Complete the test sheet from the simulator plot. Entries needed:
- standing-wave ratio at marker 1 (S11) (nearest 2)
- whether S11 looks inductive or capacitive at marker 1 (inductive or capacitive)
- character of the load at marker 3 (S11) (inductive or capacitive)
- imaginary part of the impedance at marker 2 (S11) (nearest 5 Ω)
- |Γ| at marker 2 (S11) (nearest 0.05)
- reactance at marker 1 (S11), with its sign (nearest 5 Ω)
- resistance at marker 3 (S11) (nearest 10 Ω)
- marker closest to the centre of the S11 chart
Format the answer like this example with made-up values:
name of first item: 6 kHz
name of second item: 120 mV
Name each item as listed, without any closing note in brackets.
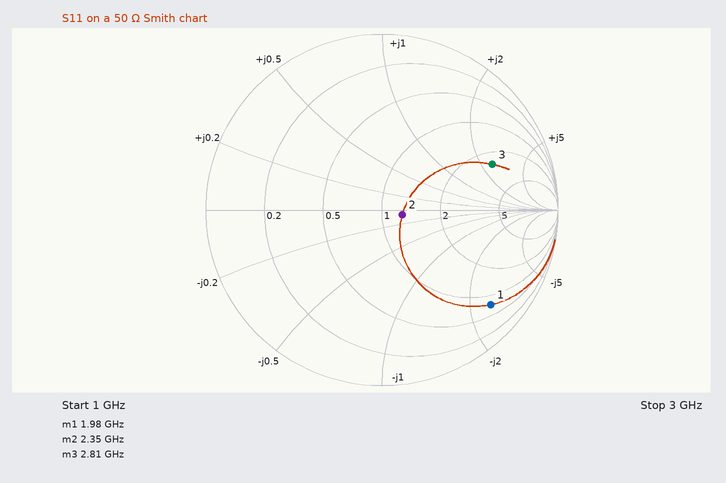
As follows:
standing-wave ratio at marker 1 (S11): 10
whether S11 looks inductive or capacitive at marker 1: capacitive
character of the load at marker 3 (S11): inductive
imaginary part of the impedance at marker 2 (S11): -5 Ω
|Γ| at marker 2 (S11): 0.10
reactance at marker 1 (S11), with its sign: -125 Ω
resistance at marker 3 (S11): 130 Ω
marker closest to the centre of the S11 chart: marker 2
